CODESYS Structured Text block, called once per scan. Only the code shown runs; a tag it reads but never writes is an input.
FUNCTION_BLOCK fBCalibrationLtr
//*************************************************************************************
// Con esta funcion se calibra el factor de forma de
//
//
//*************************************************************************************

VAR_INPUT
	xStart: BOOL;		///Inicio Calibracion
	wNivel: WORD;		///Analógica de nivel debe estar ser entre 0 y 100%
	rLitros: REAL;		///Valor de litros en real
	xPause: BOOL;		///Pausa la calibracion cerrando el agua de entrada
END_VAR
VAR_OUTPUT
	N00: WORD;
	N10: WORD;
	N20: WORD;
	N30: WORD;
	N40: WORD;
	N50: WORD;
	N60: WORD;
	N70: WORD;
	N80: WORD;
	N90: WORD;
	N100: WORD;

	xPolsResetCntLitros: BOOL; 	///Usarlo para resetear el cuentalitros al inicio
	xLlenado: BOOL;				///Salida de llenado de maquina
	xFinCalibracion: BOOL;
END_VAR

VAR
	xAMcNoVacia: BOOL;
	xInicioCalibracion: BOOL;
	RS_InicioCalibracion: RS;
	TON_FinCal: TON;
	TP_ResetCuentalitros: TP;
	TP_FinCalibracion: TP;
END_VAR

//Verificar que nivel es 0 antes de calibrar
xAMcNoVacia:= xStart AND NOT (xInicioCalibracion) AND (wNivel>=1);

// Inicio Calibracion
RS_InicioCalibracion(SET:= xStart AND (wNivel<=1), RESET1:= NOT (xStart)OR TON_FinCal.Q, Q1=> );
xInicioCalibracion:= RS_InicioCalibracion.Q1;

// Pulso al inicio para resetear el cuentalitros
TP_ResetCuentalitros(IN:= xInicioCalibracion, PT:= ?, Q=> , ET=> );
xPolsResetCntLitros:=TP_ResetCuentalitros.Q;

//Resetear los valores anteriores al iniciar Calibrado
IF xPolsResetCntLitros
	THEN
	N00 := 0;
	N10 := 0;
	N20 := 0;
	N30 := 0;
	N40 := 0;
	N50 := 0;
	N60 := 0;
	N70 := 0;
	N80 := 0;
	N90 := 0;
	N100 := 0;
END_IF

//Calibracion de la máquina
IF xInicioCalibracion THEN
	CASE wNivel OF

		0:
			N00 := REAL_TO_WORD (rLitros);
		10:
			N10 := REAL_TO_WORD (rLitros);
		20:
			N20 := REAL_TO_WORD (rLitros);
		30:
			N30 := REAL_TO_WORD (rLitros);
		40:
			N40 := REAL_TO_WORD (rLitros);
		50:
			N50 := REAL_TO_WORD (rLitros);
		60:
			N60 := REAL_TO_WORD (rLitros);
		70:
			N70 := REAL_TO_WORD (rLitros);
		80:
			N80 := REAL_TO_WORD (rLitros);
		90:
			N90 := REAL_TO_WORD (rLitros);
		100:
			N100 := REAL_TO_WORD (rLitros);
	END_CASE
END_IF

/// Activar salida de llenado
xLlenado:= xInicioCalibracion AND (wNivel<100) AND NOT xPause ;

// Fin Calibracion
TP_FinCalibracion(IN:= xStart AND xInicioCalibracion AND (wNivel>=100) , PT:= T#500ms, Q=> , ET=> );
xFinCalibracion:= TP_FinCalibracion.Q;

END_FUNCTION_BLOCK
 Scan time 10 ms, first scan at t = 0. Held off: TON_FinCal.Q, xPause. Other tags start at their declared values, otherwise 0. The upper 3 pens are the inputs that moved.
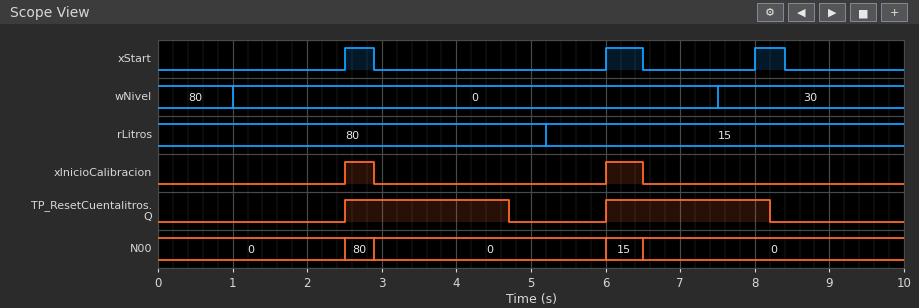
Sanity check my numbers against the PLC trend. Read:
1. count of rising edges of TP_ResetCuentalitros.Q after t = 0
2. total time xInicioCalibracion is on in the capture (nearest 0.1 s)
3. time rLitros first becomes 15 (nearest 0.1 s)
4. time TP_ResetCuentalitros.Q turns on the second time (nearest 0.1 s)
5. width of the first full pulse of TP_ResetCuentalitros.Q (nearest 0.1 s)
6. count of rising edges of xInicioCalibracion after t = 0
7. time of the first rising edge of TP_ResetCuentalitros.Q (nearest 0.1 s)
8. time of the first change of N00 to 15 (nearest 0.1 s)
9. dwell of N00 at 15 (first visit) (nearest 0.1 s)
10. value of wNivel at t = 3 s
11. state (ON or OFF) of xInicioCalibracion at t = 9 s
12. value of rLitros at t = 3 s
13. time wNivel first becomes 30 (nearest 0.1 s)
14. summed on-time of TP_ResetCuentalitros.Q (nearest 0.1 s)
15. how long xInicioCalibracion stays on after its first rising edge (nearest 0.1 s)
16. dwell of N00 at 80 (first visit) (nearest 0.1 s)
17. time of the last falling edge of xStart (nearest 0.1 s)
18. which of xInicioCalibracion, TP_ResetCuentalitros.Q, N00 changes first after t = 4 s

2
0.9 s
5.2 s
6.0 s
2.2 s
2
2.5 s
6.0 s
0.5 s
0
OFF
80
7.5 s
4.4 s
0.4 s
0.4 s
8.4 s
TP_ResetCuentalitros.Q
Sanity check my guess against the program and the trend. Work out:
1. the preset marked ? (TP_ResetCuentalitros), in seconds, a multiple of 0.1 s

2.2 s
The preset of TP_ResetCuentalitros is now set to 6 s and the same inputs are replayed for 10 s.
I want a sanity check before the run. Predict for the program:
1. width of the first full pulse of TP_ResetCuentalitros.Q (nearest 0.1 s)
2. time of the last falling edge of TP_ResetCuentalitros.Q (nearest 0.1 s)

6.0 s
8.5 s
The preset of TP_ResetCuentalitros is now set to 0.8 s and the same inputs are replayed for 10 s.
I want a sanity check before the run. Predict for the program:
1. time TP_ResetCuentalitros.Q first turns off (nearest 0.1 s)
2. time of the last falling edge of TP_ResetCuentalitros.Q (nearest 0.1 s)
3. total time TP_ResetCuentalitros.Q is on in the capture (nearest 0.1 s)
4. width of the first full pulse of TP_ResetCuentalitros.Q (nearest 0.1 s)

3.3 s
6.8 s
1.6 s
0.8 s
